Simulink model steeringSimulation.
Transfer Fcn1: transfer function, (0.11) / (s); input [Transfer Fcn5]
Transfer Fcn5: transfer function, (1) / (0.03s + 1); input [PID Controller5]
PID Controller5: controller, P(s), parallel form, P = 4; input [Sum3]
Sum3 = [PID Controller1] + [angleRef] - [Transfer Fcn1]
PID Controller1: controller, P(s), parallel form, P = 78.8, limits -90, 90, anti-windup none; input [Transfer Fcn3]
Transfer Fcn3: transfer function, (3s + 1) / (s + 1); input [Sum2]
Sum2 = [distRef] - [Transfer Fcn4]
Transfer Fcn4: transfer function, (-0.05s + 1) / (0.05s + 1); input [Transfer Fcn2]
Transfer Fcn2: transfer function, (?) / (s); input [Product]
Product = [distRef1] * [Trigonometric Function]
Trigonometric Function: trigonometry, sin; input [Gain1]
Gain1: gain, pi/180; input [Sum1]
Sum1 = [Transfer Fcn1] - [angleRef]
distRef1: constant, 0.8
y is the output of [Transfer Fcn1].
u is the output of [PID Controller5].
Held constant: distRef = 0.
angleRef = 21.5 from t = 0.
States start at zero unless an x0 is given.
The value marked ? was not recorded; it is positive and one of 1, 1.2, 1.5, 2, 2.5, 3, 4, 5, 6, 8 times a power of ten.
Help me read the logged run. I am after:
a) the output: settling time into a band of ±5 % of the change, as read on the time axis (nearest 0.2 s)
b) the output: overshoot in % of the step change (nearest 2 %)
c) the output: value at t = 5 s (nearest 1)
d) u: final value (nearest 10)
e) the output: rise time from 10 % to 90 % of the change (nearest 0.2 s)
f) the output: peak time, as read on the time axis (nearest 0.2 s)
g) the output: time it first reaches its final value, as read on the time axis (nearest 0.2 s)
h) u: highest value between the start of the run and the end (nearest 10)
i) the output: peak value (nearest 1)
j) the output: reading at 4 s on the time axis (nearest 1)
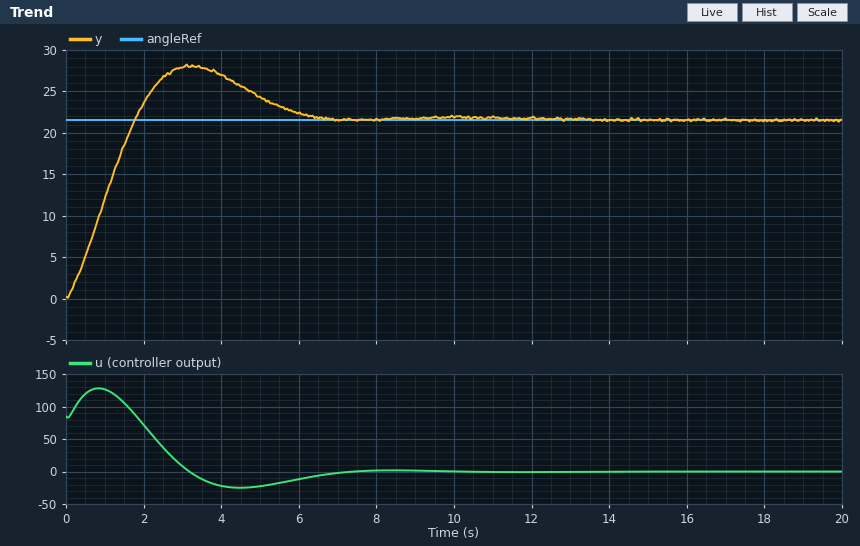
5.8 s
30 %
24
0
1.4 s
3.2 s
1.8 s
130
28
27
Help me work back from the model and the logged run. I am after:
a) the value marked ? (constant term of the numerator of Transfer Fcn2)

0.6
